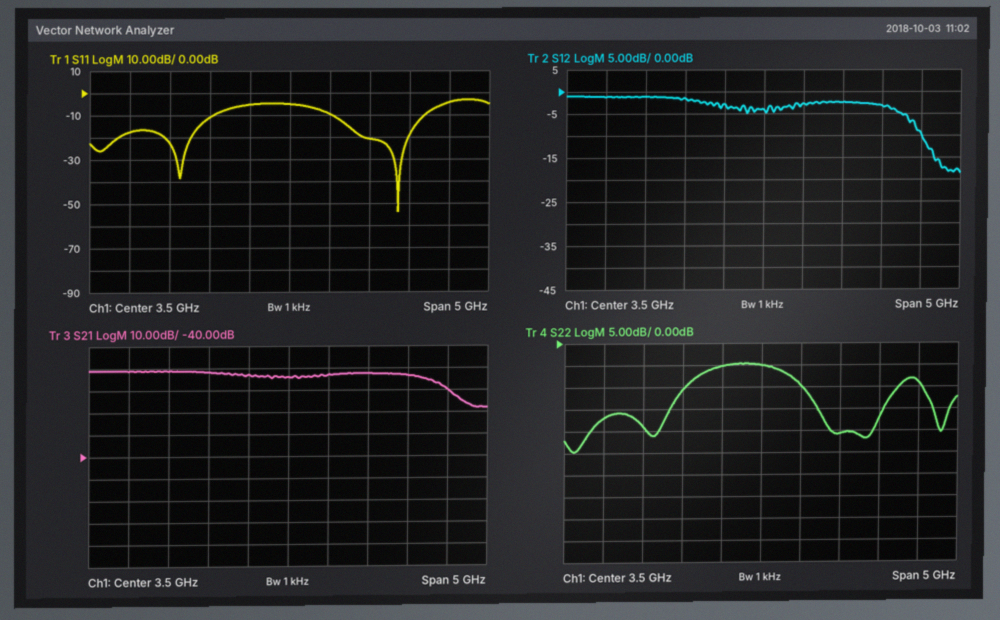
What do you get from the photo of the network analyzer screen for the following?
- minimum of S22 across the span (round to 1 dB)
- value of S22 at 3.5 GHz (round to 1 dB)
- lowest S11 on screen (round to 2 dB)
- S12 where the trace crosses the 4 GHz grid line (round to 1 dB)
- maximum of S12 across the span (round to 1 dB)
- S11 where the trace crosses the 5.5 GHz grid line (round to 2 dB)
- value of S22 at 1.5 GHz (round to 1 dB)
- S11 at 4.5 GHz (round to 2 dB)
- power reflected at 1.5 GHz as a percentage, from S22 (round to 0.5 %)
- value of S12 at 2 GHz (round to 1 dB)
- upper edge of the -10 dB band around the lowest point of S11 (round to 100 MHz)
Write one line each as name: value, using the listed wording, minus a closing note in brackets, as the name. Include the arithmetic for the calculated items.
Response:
minimum of S22 across the span: -25 dB
value of S22 at 3.5 GHz: -5 dB
lowest S11 on screen: -54 dB
S12 where the trace crosses the 4 GHz grid line: -3 dB
maximum of S12 across the span: -1 dB
S11 where the trace crosses the 5.5 GHz grid line: -4 dB
value of S22 at 1.5 GHz: -17 dB
S11 at 4.5 GHz: -20 dB
power reflected at 1.5 GHz as a percentage, from S22: 10^(-17/10) ≈ 2.0 %
value of S12 at 2 GHz: -1 dB
upper edge of the -10 dB band around the lowest point of S11: 5.2 GHz
